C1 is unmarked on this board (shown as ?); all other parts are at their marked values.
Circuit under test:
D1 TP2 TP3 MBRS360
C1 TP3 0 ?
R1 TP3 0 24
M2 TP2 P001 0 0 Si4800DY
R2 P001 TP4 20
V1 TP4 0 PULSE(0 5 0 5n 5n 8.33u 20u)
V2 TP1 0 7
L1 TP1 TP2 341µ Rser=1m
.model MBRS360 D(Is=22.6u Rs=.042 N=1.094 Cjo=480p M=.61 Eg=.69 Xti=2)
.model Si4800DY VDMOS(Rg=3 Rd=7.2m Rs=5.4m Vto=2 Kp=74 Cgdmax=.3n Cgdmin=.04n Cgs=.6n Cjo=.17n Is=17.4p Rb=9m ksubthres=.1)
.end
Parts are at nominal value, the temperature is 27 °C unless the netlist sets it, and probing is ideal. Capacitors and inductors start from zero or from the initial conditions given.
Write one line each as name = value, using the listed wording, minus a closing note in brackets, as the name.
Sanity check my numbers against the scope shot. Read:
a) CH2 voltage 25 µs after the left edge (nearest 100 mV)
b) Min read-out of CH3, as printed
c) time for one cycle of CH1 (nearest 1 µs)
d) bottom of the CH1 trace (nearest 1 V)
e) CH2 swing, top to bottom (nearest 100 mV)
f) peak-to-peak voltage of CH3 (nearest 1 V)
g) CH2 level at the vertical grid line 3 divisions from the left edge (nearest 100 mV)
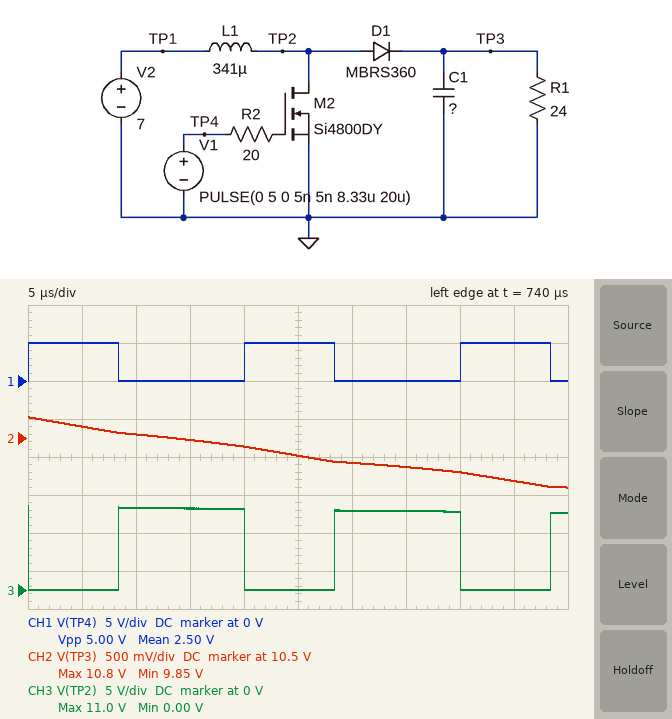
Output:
CH2 voltage 25 µs after the left edge = 10.3 V
Min read-out of CH3, as printed = 0.00 V
time for one cycle of CH1 = 20 µs
bottom of the CH1 trace = 0 V
CH2 swing, top to bottom = 900 mV
peak-to-peak voltage of CH3 = 11 V
CH2 level at the vertical grid line 3 divisions from the left edge = 10.5 V
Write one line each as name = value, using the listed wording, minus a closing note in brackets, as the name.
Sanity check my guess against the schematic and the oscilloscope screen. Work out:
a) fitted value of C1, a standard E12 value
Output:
fitted value of C1, a standard E12 value = 18 µF
